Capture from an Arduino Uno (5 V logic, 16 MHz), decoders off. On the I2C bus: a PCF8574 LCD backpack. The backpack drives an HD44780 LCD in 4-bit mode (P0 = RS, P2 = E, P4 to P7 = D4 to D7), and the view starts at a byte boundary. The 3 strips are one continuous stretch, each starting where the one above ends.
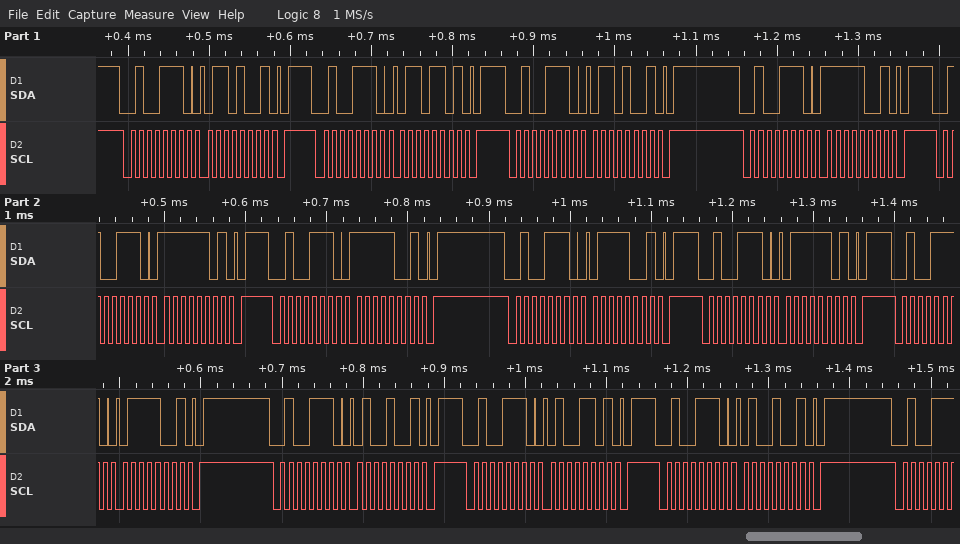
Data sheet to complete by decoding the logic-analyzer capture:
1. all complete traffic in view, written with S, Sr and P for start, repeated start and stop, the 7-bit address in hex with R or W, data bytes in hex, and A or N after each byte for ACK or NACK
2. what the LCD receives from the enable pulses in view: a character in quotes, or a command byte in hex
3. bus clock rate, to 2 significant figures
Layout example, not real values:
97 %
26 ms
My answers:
S 27W A 69 A P S 27W A 6D A P S 27W A 69 A P S 27W A F9 A P S 27W A FD A P S 27W A F9 A P S 27W A 79 A P S 27W A 7D A P S 27W A 79 A P S 27W A 49 A P S 27W A 4D A P S 27W A 49 A P
'o' 't'
100 kHz
